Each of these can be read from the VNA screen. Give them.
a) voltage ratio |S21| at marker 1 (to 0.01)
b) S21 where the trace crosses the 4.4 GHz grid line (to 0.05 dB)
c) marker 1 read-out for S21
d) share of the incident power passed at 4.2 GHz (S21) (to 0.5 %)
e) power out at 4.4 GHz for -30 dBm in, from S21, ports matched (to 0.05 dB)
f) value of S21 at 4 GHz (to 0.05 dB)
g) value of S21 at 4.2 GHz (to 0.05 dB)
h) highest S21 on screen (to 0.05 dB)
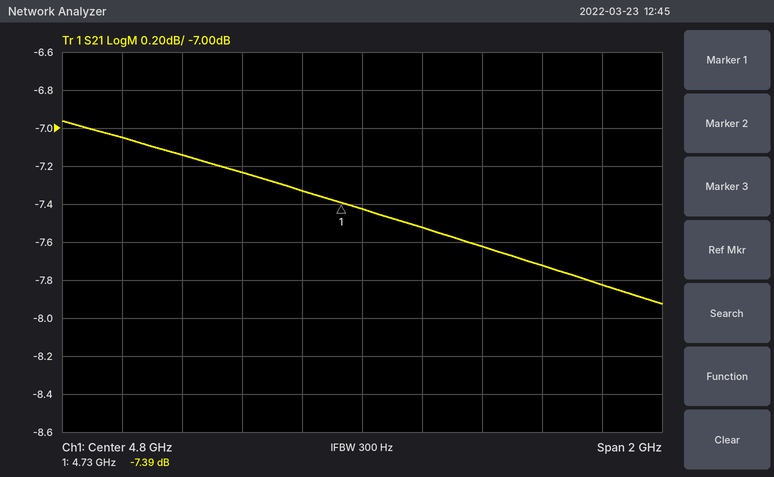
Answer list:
0.43
-7.25 dB
-7.39 dB
19.5 %
-37.25 dBm
-7.05 dB
-7.15 dB
-6.95 dB
